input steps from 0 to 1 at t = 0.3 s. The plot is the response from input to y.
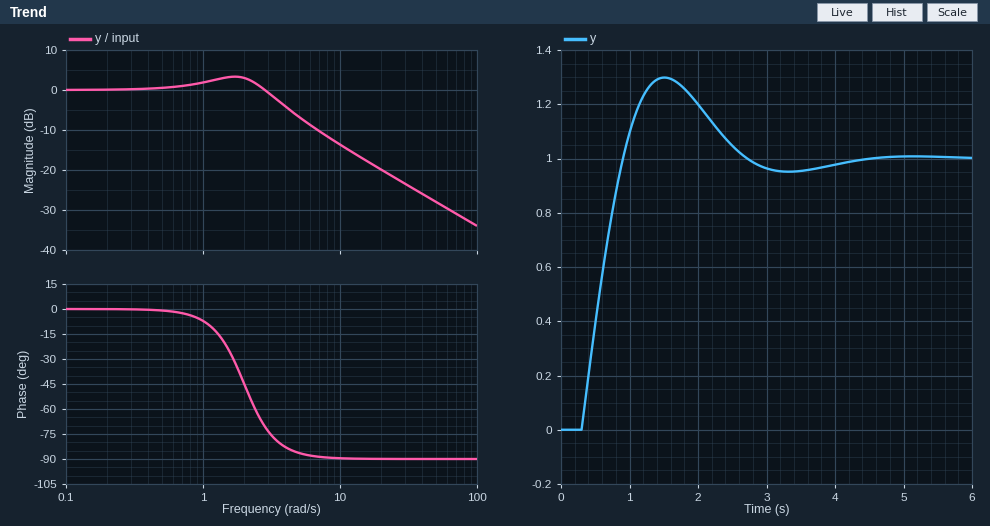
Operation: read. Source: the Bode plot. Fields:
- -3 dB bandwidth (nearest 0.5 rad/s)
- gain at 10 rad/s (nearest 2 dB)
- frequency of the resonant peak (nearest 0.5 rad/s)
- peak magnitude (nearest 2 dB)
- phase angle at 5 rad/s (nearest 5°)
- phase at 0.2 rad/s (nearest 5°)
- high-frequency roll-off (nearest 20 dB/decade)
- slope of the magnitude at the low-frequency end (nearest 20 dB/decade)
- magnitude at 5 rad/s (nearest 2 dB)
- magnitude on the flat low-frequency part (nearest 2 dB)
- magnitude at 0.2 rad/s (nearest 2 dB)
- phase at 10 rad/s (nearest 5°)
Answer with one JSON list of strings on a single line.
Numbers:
["3.5 rad/s", "-14 dB", "1.5 rad/s", "4 dB", "-85°", "0°", "-20 dB/decade", "0 dB/decade", "-6 dB", "0 dB", "0 dB", "-90°"]
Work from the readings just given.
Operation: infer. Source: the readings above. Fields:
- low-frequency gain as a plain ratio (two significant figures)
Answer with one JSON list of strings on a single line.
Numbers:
["1.0"]
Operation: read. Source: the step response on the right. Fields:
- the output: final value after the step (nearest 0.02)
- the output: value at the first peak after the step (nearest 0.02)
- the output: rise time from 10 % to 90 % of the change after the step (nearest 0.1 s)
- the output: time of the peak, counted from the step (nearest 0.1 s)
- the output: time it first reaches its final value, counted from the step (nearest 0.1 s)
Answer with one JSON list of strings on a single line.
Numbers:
["1.00", "1.30", "0.5 s", "1.2 s", "0.6 s"]
